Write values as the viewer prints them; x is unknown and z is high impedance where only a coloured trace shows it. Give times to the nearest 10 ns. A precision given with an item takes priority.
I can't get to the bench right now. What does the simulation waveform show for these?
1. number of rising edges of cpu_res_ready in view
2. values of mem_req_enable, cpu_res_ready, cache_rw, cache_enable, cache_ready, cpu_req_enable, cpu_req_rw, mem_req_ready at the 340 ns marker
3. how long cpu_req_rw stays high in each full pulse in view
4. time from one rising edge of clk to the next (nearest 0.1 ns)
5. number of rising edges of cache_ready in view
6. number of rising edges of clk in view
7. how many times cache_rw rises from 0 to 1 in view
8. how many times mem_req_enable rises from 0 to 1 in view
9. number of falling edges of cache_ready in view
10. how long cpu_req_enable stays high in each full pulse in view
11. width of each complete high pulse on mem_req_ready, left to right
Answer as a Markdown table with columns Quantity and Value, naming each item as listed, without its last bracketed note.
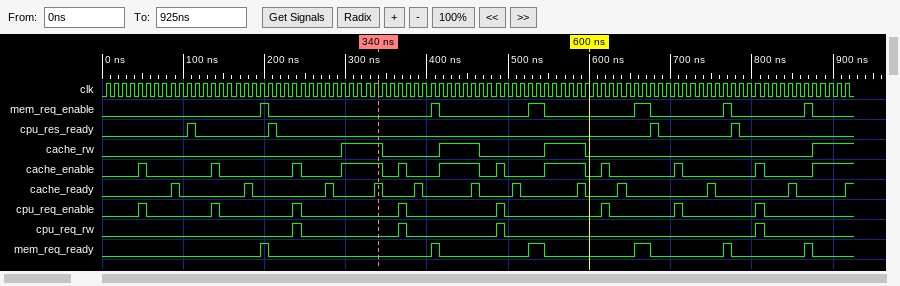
| Quantity | Value |
|---|---|
| number of rising edges of cpu_res_ready in view | 4 |
| values of mem_req_enable, cpu_res_ready, cache_rw, cache_enable, cache_ready, cpu_req_enable, cpu_req_rw, mem_req_ready at the 340 ns marker | mem_req_enable=0, cpu_res_ready=0, cache_rw=1, cache_enable=1, cache_ready=1, cpu_req_enable=0, cpu_req_rw=0, mem_req_ready=0 |
| how long cpu_req_rw stays high in each full pulse in view | 10 ns, 10 ns, 10 ns, 10 ns |
| time from one rising edge of clk to the next | 10 ns |
| number of rising edges of cache_ready in view | 12 |
| number of rising edges of clk in view | 92 |
| how many times cache_rw rises from 0 to 1 in view | 4 |
| how many times mem_req_enable rises from 0 to 1 in view | 6 |
| number of falling edges of cache_ready in view | 11 |
| how long cpu_req_enable stays high in each full pulse in view | 10 ns, 10 ns, 10 ns, 10 ns, 10 ns, 10 ns, 10 ns, 10 ns |
| width of each complete high pulse on mem_req_ready, left to right | 10 ns, 10 ns, 20 ns, 20 ns, 10 ns, 10 ns |
